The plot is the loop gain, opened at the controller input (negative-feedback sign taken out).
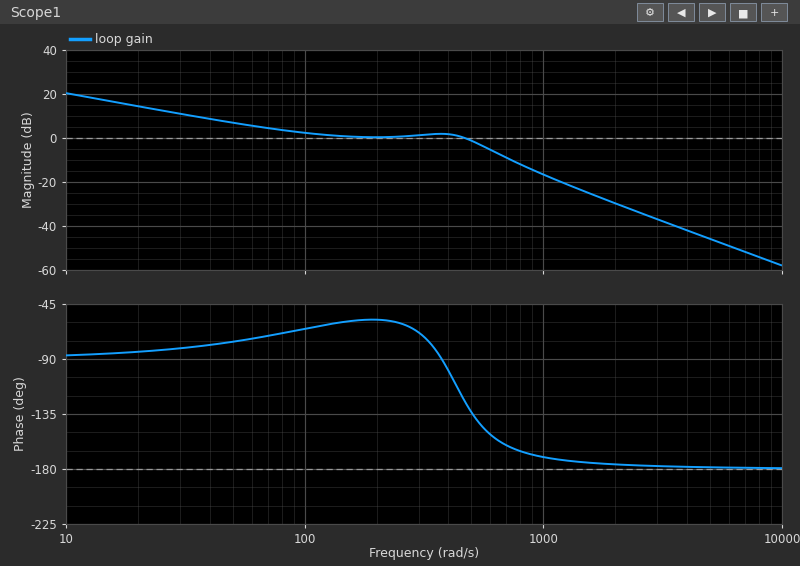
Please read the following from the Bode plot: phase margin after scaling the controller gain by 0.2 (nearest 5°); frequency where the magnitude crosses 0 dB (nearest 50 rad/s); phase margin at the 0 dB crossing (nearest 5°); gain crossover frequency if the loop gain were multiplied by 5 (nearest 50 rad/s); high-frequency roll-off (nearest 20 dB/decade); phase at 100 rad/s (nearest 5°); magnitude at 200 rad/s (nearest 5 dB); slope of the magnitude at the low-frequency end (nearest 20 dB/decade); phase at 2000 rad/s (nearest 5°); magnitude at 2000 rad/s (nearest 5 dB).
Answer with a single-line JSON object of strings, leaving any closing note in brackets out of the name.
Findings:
{"phase margin after scaling the controller gain by 0.2": "95°", "frequency where the magnitude crosses 0 dB": "450 rad/s", "phase margin at the 0 dB crossing": "55°", "gain crossover frequency if the loop gain were multiplied by 5": "900 rad/s", "high-frequency roll-off": "-40 dB/decade", "phase at 100 rad/s": "-65°", "magnitude at 200 rad/s": "0 dB", "slope of the magnitude at the low-frequency end": "-20 dB/decade", "phase at 2000 rad/s": "-175°", "magnitude at 2000 rad/s": "-30 dB"}
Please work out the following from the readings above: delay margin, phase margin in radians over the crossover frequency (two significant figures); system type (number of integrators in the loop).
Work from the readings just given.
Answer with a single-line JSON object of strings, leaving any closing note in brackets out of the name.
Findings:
{"delay margin, phase margin in radians over the crossover frequency": "0.0021 s", "system type": "1"}
